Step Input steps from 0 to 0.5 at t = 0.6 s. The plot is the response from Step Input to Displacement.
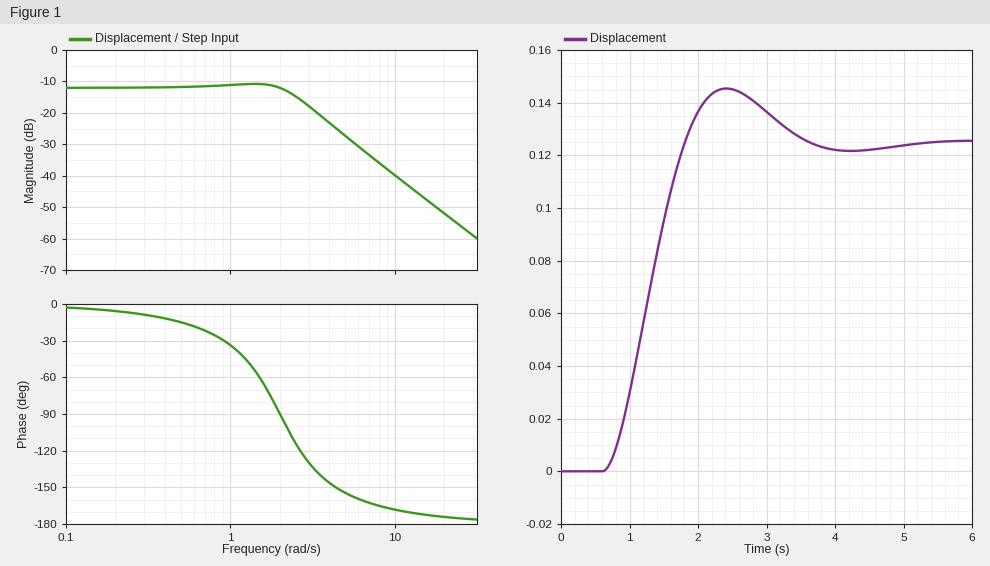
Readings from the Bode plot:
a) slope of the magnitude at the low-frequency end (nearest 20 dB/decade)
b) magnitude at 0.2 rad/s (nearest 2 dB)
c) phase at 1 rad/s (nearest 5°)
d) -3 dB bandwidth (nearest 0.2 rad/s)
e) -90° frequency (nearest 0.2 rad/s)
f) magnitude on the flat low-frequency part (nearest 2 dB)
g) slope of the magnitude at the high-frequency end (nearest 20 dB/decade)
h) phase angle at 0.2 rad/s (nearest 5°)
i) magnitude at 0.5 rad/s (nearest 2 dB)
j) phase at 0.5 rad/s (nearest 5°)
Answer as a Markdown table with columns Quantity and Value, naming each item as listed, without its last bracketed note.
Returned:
| Quantity | Value |
|---|---|
| slope of the magnitude at the low-frequency end | 0 dB/decade |
| magnitude at 0.2 rad/s | -12 dB |
| phase at 1 rad/s | -35° |
| -3 dB bandwidth | 2.6 rad/s |
| -90° frequency | 2.0 rad/s |
| magnitude on the flat low-frequency part | -12 dB |
| slope of the magnitude at the high-frequency end | -40 dB/decade |
| phase angle at 0.2 rad/s | -5° |
| magnitude at 0.5 rad/s | -12 dB |
| phase at 0.5 rad/s | -15° |
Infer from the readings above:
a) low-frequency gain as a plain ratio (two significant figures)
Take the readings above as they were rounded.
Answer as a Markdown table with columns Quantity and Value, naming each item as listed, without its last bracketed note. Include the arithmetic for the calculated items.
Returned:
| Quantity | Value |
|---|---|
| low-frequency gain as a plain ratio | 10^(-12 / 20) = 0.25 |
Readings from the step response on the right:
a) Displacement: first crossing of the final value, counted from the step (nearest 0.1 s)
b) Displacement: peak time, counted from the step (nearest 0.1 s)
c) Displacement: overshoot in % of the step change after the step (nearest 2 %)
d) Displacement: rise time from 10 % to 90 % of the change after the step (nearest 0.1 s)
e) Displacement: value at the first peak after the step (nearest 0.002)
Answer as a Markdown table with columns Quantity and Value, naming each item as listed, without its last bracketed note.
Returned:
| Quantity | Value |
|---|---|
| Displacement: first crossing of the final value, counted from the step | 1.2 s |
| Displacement: peak time, counted from the step | 1.8 s |
| Displacement: overshoot in % of the step change after the step | 16 % |
| Displacement: rise time from 10 % to 90 % of the change after the step | 0.8 s |
| Displacement: value at the first peak after the step | 0.146 |
